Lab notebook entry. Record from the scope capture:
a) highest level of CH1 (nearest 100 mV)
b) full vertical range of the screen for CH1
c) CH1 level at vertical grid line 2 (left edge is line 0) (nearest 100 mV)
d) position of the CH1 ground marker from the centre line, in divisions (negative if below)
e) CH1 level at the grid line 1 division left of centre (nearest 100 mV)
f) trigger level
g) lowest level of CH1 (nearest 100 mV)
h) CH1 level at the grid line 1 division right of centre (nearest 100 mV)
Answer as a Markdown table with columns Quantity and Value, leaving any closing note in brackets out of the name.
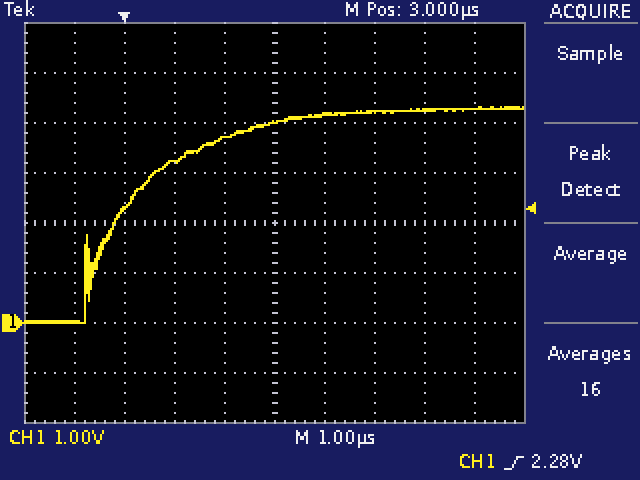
| Quantity | Value |
|---|---|
| highest level of CH1 | 4.3 V |
| full vertical range of the screen for CH1 | 8 V |
| CH1 level at vertical grid line 2 (left edge is line 0) | 2.3 V |
| position of the CH1 ground marker from the centre line, in divisions | -2.0 div |
| CH1 level at the grid line 1 division left of centre | 3.7 V |
| trigger level | 2.28 V |
| lowest level of CH1 | 0.0 V |
| CH1 level at the grid line 1 division right of centre | 4.2 V |
